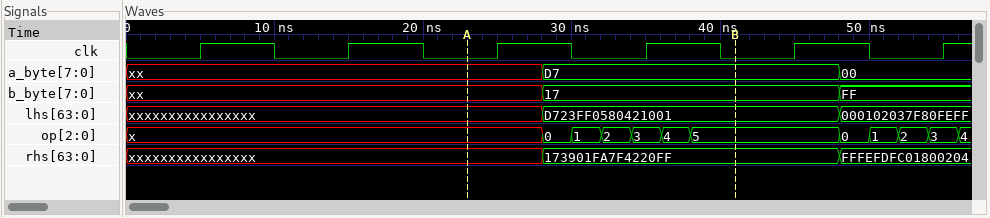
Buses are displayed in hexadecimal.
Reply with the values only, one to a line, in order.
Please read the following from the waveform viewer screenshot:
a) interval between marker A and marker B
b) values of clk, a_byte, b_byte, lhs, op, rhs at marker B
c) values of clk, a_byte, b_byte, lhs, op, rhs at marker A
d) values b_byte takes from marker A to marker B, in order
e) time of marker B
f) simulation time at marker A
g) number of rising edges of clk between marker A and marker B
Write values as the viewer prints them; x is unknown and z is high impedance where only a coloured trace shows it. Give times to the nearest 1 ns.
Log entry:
18 ns
clk=0, a_byte=D7, b_byte=17, lhs=D723FF0580421001, op=5, rhs=173901FA7F4220FF
clk=0, a_byte=xx, b_byte=xx, lhs=xxxxxxxxxxxxxxxx, op=x, rhs=xxxxxxxxxxxxxxxx
xx, 17
41 ns
23 ns
2
